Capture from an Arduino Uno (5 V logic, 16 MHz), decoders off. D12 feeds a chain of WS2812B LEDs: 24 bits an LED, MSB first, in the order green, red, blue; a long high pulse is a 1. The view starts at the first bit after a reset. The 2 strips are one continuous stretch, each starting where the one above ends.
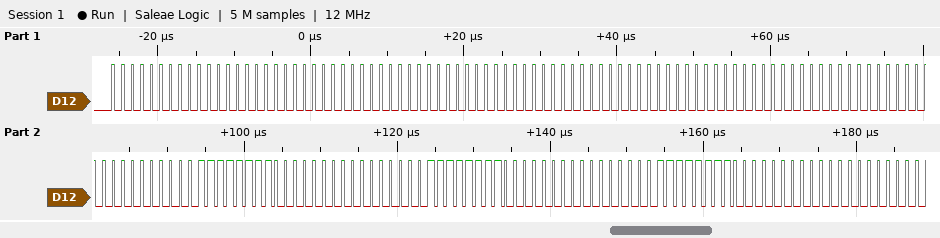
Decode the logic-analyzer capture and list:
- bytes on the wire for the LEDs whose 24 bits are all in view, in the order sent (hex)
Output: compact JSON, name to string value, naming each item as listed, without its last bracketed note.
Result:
{"bytes on the wire for the LEDs whose 24 bits are all in view, in the order sent": "00 00 00 00 00 00 00 00 00 00 00 00 FF 00 00 FF 00 00 FF 00 00"}
